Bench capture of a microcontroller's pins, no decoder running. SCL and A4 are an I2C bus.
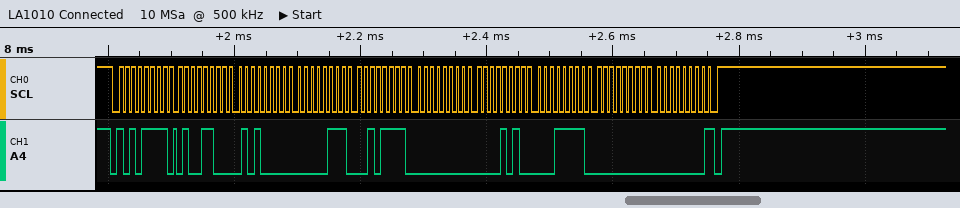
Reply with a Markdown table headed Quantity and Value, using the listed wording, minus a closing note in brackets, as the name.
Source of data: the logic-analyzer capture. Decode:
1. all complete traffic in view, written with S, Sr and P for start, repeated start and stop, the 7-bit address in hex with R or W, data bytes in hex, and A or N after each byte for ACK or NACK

| Quantity | Value |
|---|---|
| all complete traffic in view, written with S, Sr and P for start, repeated start and stop, the 7-bit address in hex with R or W, data bytes in hex, and A or N after each byte for ACK or NACK | S 57R A 4C A 50 A 07 A 2F A 00 A 0A A 1F A 00 A 00 N P |
